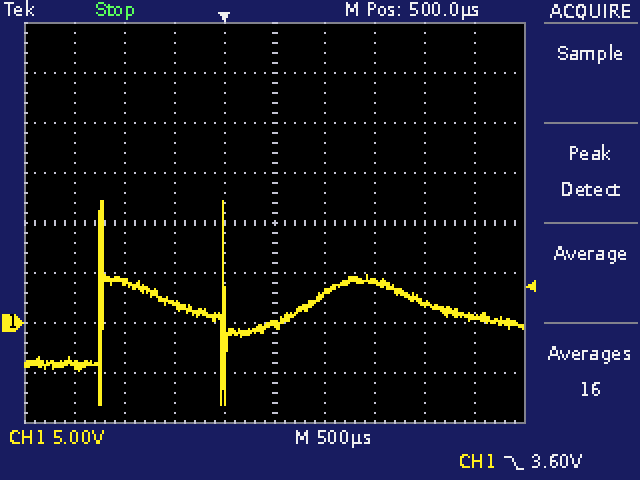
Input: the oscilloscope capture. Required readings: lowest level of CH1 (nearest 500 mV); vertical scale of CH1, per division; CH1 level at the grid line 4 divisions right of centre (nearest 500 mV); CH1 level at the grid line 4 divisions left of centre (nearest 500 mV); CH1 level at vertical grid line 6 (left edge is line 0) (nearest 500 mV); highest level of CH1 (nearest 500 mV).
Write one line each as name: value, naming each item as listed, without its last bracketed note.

lowest level of CH1: -8.0 V
vertical scale of CH1, per division: 5 V
CH1 level at the grid line 4 divisions right of centre: 500 mV
CH1 level at the grid line 4 divisions left of centre: -4.0 V
CH1 level at vertical grid line 6 (left edge is line 0): 3.0 V
highest level of CH1: 12.0 V
